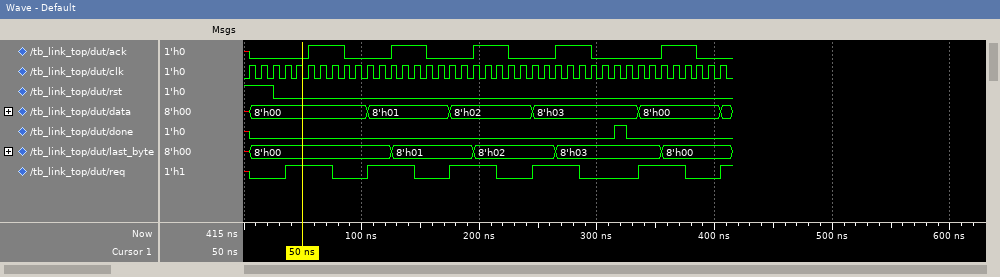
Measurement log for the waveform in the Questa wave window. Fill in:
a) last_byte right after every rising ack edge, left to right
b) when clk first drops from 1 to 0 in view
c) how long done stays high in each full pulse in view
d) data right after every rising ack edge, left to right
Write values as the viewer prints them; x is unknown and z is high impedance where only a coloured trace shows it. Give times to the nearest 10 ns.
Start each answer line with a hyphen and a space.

- 8'h00, 8'h01, 8'h02, 8'h03, 8'h00
- 10 ns
- 10 ns
- 8'h00, 8'h01, 8'h02, 8'h03, 8'h00
